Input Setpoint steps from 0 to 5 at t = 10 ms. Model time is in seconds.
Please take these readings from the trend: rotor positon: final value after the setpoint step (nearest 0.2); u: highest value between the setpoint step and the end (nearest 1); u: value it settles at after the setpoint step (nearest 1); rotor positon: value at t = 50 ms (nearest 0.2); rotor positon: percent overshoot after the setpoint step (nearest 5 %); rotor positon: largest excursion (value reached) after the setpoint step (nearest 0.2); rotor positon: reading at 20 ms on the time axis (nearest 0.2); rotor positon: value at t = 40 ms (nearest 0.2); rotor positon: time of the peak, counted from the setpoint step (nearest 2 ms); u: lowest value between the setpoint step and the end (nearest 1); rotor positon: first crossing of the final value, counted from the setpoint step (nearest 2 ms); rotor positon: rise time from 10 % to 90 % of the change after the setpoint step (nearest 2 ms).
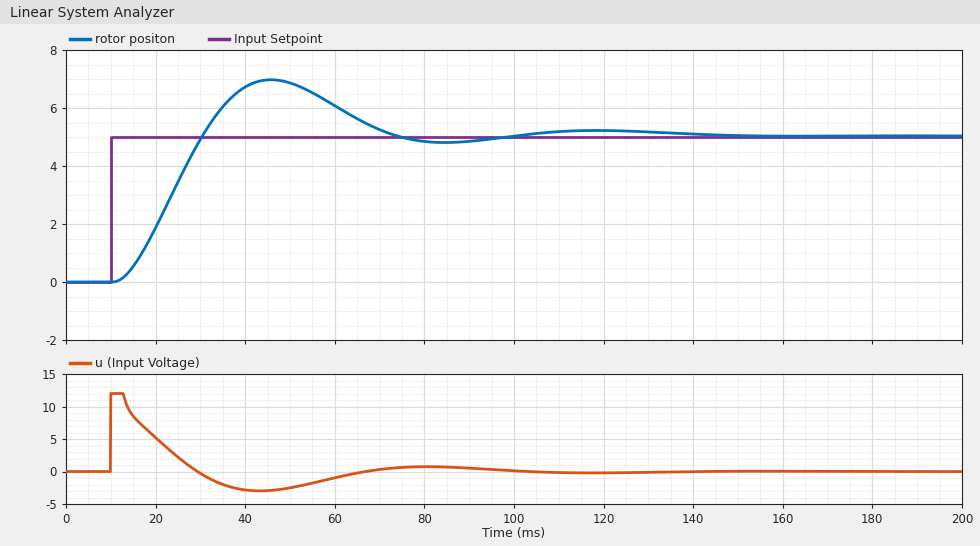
5.0
12
0
6.8
40 %
7.0
1.8
6.8
36 ms
-3
20 ms
14 ms
